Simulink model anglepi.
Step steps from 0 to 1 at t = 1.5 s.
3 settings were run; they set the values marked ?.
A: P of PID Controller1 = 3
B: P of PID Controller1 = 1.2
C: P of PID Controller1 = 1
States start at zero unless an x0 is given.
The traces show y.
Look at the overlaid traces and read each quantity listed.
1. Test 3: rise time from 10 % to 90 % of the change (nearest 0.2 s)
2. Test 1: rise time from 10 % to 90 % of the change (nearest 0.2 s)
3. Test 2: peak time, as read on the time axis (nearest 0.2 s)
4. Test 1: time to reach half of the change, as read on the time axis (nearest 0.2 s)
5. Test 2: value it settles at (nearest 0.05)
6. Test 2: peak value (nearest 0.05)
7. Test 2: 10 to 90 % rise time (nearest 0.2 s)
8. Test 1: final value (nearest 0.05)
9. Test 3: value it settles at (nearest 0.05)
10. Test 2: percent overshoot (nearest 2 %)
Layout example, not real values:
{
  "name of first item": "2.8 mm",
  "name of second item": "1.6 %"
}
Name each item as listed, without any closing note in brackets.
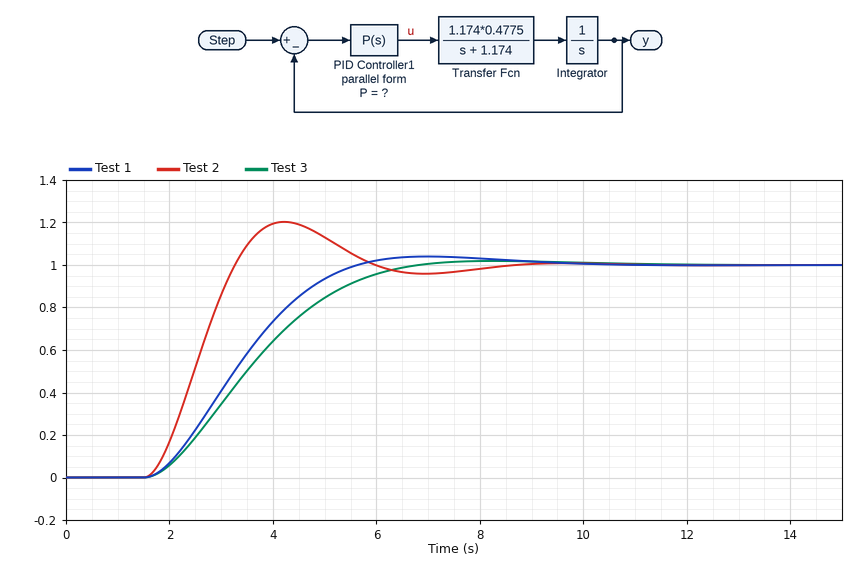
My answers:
{
  "Test 3: rise time from 10 % to 90 % of the change": "3.2 s",
  "Test 1: rise time from 10 % to 90 % of the change": "2.6 s",
  "Test 2: peak time, as read on the time axis": "4.2 s",
  "Test 1: time to reach half of the change, as read on the time axis": "3.2 s",
  "Test 2: value it settles at": "1.00",
  "Test 2: peak value": "1.20",
  "Test 2: 10 to 90 % rise time": "1.2 s",
  "Test 1: final value": "1.00",
  "Test 3: value it settles at": "1.00",
  "Test 2: percent overshoot": "20 %"
}
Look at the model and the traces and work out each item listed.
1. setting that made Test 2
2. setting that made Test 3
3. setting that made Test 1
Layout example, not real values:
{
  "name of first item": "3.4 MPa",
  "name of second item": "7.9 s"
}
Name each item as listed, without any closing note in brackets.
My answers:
{
  "setting that made Test 2": "A",
  "setting that made Test 3": "C",
  "setting that made Test 1": "B"
}
